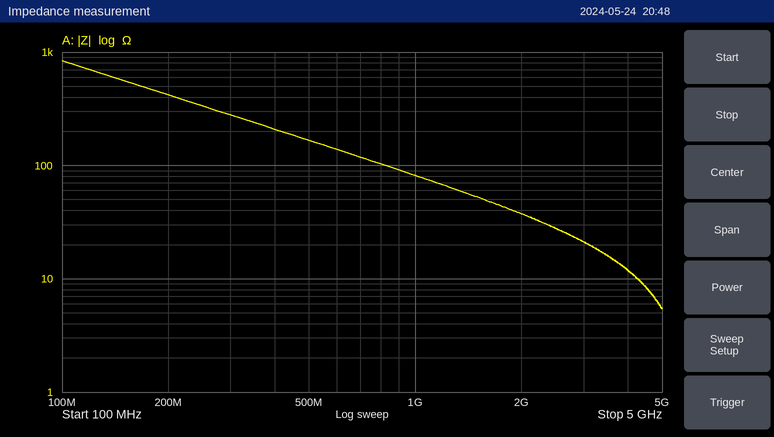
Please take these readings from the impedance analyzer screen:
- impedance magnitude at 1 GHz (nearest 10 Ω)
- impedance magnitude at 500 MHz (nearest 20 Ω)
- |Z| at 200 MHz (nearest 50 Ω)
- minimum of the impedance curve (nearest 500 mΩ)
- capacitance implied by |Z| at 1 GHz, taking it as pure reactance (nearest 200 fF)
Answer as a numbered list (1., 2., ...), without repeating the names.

1. 80 Ω
2. 160 Ω
3. 400 Ω
4. 5.5 Ω
5. 2.0 pF
